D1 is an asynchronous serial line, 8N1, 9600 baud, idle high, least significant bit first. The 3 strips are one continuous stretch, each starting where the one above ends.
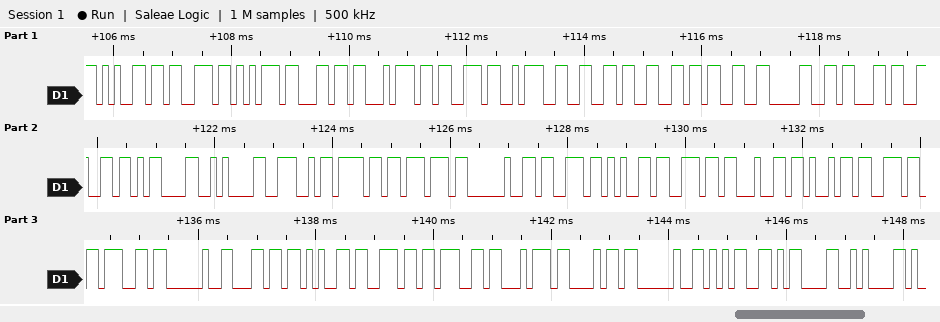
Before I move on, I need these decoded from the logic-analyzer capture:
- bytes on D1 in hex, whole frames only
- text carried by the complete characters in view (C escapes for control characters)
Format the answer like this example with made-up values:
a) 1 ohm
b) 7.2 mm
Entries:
a) 65 73 75 6C 74 73 3A 66 66 33 30 63 66 0D 0A 4E 6F 77 20 73 65 6E 64 69 6E 67 20 6C 65 6E 67 74 68 20 35 0D 0A
b) "esults:ff30cf\r\nNow sending length 5\r\n"
